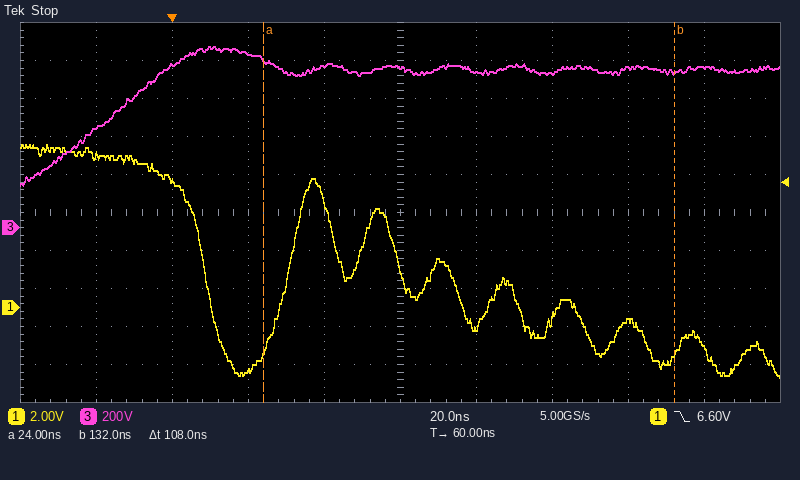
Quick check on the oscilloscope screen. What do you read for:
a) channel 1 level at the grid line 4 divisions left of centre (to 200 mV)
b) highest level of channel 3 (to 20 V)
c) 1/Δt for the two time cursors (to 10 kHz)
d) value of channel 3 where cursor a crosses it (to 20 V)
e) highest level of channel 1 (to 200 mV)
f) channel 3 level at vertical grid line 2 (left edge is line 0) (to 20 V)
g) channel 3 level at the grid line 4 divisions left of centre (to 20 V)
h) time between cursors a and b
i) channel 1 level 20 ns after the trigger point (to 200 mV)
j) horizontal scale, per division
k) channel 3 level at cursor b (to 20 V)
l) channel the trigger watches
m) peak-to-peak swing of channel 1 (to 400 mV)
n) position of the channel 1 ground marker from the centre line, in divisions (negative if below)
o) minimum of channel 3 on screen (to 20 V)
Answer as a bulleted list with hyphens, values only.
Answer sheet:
- 8.0 V
- 960 V
- 9.26 MHz
- 880 V
- 8.6 V
- 860 V
- 520 V
- 108 ns
- -3.4 V
- 20 ns
- 820 V
- channel 1
- 12.4 V
- -2.5 div
- 220 V
